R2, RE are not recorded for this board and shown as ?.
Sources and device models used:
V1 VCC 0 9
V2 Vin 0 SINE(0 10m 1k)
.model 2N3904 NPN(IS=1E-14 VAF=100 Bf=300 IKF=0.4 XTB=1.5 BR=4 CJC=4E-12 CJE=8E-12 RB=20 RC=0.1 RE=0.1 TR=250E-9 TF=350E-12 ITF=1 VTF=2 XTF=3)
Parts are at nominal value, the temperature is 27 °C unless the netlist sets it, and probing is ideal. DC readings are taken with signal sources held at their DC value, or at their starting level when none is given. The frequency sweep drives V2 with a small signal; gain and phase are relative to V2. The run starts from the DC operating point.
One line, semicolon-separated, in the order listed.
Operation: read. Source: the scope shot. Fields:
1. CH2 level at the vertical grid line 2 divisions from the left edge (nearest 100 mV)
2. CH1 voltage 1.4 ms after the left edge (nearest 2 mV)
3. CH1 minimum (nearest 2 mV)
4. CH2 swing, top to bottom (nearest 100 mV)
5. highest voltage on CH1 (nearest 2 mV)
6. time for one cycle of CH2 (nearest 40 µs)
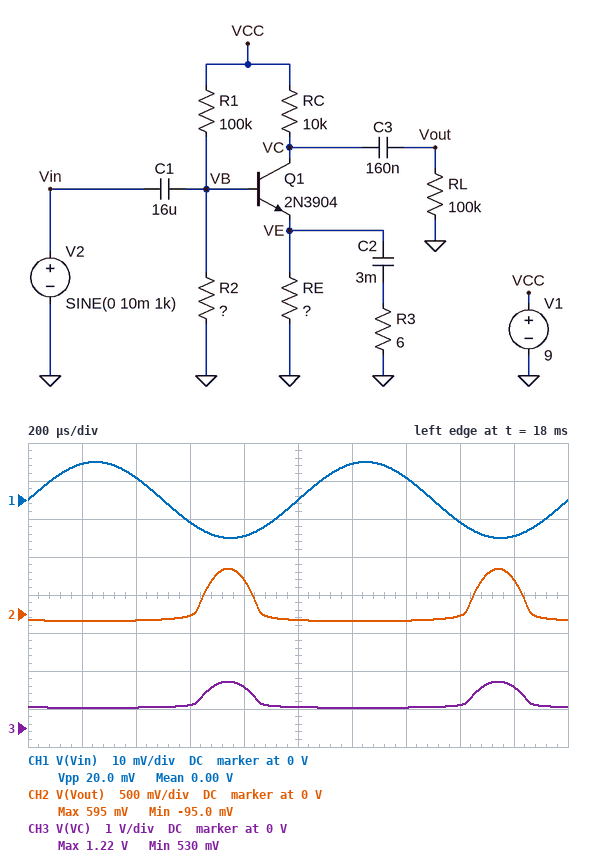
-100 mV; 6 mV; -10 mV; 700 mV; 10 mV; 1.00 ms
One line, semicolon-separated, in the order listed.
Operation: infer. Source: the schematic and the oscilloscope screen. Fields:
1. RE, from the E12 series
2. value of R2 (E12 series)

560 Ω; 47 kΩ
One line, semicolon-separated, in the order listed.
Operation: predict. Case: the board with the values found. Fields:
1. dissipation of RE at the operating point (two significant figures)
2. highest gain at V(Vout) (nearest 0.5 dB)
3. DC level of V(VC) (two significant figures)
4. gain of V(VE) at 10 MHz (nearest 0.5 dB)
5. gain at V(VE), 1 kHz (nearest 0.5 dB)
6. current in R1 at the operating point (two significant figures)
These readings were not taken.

450 µW; 8.5 dB; 550 mV; -18.5 dB; -27.5 dB; 78 µA
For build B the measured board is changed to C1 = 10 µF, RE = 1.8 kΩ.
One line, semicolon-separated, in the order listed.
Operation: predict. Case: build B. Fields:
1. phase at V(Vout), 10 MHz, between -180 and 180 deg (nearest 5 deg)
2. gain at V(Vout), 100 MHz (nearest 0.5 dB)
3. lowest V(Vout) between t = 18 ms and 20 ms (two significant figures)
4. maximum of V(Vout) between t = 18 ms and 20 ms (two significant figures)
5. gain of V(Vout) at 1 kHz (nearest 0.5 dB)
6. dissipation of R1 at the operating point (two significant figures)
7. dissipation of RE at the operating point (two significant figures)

25 deg; -4.0 dB; -340 mV; 1.3 V; 14.5 dB; 480 µW; 1.1 mW
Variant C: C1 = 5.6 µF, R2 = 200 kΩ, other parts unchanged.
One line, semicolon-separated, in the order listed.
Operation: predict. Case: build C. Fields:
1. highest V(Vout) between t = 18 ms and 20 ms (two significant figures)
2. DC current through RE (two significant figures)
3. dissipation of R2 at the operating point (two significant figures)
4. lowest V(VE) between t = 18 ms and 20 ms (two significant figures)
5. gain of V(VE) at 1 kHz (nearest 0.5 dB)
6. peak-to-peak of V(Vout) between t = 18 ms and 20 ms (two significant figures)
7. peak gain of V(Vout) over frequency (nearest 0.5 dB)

66 mV; 920 µA; 6.9 µW; 510 mV; -27.0 dB; 87 mV; 5.5 dB
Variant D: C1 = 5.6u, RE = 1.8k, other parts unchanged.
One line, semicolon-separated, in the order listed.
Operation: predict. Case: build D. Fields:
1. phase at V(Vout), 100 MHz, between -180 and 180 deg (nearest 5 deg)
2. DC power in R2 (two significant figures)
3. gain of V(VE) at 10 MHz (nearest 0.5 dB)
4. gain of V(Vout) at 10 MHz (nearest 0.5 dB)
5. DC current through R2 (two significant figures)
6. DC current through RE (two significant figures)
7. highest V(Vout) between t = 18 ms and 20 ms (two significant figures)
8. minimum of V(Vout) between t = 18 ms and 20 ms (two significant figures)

-5 deg; 90 µW; -19.5 dB; -3.0 dB; 44 µA; 780 µA; 1.3 V; -340 mV
